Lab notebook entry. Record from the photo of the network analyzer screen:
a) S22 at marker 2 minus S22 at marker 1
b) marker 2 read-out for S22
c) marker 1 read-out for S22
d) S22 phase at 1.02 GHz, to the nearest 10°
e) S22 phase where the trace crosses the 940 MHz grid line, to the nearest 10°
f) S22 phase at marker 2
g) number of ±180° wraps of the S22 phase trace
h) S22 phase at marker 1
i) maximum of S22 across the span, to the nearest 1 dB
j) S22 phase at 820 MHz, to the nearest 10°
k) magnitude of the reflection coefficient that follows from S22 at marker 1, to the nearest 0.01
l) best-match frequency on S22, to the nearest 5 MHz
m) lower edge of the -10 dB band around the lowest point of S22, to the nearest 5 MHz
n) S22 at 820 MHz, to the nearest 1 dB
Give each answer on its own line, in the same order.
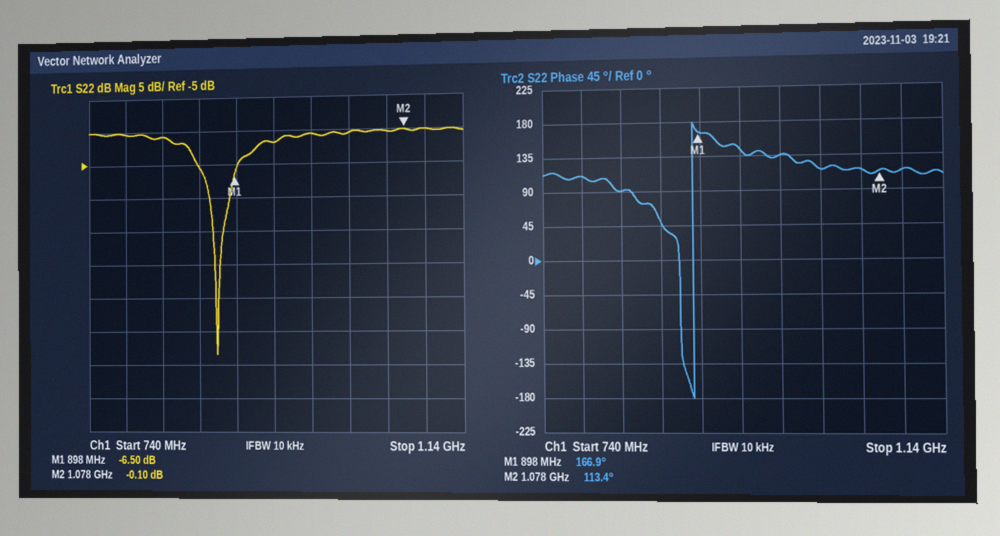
6.40 dB
-0.10 dB
-6.50 dB
120°
140°
113.4°
1
166.9°
0 dB
90°
0.47
880 MHz
870 MHz
-1 dB
